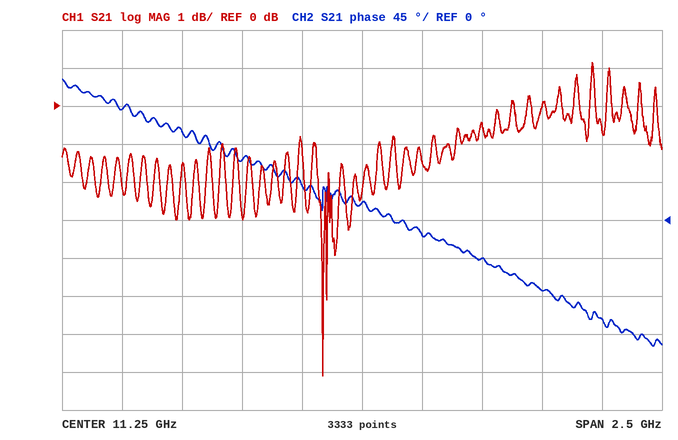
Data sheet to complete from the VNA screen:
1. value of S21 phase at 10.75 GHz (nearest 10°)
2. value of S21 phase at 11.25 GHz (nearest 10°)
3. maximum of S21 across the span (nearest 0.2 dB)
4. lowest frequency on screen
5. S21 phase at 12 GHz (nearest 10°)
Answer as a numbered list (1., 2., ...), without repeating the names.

1. 70°
2. 20°
3. 1.2 dB
4. 10 GHz
5. -80°
